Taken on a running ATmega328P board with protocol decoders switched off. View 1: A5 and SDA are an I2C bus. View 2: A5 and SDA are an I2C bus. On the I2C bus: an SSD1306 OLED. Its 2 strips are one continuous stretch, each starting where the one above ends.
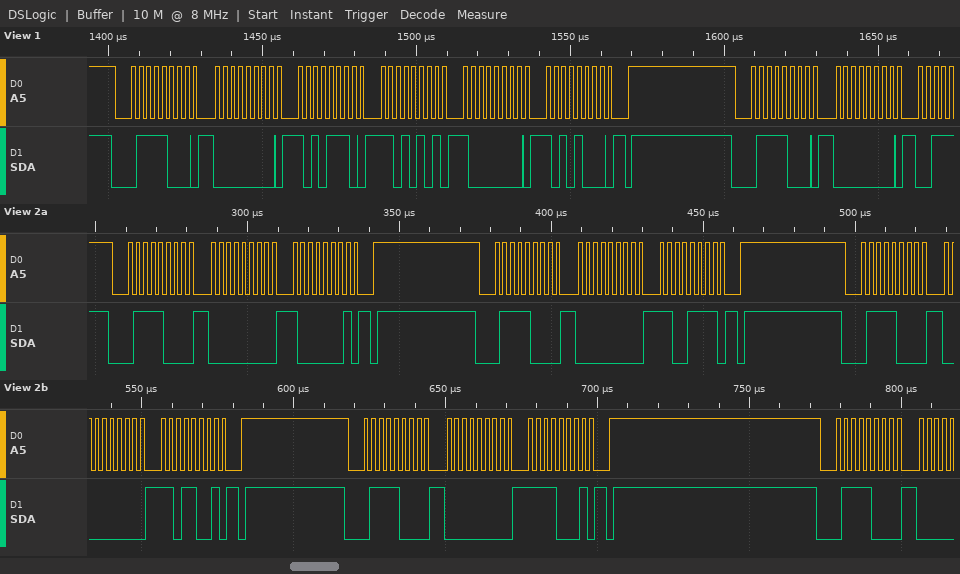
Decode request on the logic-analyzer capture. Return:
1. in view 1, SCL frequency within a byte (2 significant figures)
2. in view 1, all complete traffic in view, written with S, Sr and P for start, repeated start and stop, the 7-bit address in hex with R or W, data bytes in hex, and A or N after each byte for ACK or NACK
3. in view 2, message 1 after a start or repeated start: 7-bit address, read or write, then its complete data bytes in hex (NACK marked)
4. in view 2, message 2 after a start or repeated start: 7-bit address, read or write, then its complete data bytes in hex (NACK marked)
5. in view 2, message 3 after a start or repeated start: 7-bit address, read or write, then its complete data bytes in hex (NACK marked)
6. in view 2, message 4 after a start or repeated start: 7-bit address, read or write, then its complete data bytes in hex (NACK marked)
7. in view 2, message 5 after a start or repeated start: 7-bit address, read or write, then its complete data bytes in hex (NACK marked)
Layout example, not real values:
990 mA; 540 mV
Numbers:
400 kHz; S 3CW A 00 A AE A D5 A 80 A A8 A P S 3CW A 00 A; 0x3C write: 00 81; 0x3C write: 00 CF; 0x3C write: 00 D9; 0x3C write: 00 F1; 0x3C write
